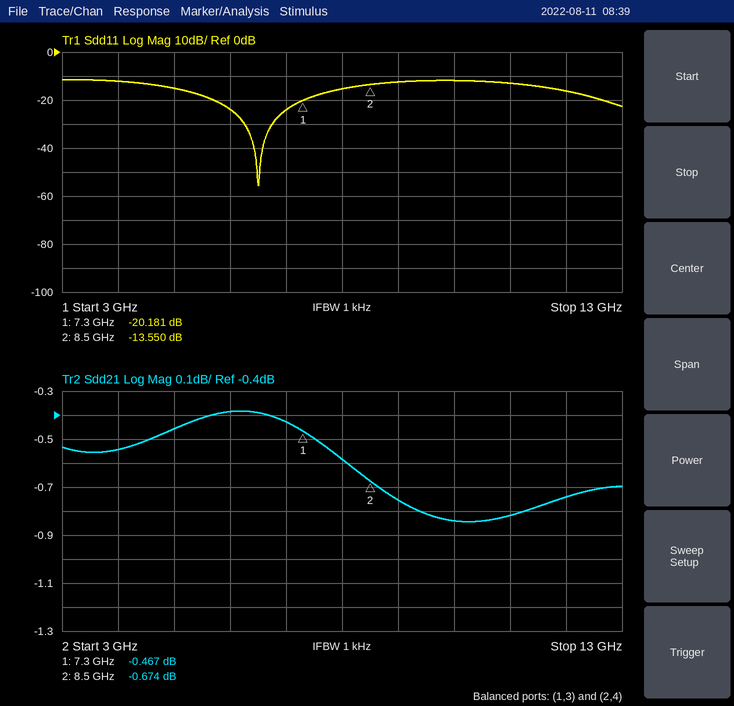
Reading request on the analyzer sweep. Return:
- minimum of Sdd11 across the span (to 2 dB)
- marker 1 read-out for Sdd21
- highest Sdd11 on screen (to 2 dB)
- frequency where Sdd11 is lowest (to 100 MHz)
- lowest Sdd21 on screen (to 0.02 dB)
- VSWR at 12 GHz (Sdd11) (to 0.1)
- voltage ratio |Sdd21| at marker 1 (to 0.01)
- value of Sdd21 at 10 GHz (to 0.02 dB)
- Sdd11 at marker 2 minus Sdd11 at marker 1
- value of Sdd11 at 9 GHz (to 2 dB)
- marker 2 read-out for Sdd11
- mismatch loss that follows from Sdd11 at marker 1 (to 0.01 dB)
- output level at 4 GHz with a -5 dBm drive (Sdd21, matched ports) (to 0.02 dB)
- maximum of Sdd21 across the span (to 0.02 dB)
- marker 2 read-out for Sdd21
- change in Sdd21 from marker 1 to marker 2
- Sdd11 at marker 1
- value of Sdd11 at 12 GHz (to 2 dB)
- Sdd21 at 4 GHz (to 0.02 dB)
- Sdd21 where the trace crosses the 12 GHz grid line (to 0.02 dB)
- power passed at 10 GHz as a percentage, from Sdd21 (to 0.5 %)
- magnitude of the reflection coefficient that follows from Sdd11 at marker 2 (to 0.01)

-56 dB
-0.467 dB
-12 dB
6.5 GHz
-0.84 dB
1.4
0.95
-0.84 dB
6.631 dB
-12 dB
-13.550 dB
0.04 dB
-5.54 dBm
-0.38 dB
-0.674 dB
-0.207 dB
-20.181 dB
-16 dB
-0.54 dB
-0.74 dB
82.5 %
0.21
